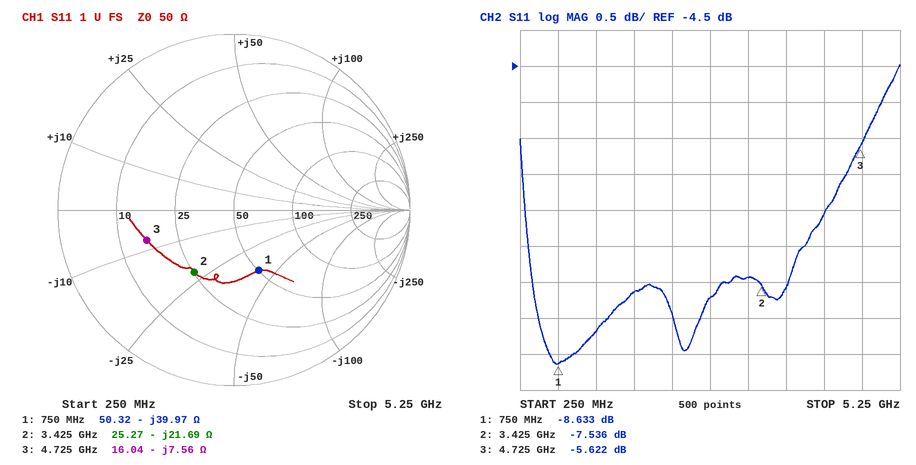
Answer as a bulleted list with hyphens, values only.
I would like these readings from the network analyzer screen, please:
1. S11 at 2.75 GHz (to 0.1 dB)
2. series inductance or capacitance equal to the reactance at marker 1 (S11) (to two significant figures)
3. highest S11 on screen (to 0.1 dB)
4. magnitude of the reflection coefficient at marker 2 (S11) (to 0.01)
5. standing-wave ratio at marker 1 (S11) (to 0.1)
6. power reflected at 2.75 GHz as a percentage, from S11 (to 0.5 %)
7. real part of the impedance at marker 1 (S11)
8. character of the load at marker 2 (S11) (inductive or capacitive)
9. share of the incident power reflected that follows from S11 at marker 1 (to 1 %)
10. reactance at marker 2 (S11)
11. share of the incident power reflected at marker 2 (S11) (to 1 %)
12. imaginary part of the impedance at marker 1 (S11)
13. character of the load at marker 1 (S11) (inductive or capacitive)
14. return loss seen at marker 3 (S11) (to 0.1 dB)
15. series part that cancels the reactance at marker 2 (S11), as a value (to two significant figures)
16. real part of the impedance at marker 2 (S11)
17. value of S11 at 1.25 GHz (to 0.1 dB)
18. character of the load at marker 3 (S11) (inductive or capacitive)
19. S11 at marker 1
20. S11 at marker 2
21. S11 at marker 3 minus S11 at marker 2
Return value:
- -7.7 dB
- 5.3 pF
- -4.5 dB
- 0.42
- 2.2
- 17.0 %
- 50.32 Ω
- capacitive
- 14 %
- -21.69 Ω
- 18 %
- -39.97 Ω
- capacitive
- 5.6 dB
- 1.0 nH
- 25.27 Ω
- -8.2 dB
- capacitive
- -8.633 dB
- -7.536 dB
- 1.914 dB
